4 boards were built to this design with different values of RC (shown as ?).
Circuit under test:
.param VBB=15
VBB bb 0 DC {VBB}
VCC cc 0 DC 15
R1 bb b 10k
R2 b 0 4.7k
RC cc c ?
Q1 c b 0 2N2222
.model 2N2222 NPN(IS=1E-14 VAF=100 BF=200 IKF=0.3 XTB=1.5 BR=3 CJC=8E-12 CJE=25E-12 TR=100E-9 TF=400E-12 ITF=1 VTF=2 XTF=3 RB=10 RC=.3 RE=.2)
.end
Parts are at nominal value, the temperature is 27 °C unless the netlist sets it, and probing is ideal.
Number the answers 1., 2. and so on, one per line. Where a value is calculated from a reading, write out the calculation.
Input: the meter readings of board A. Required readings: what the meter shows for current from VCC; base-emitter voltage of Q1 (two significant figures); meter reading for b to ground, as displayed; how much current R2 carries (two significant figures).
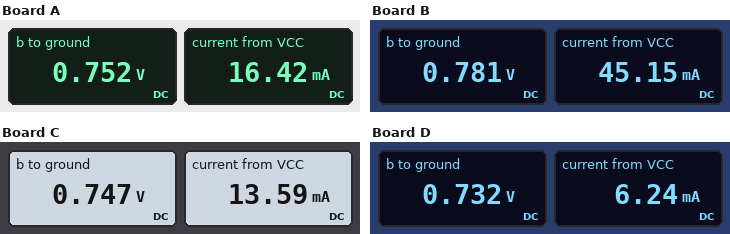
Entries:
1. 16.42 mA
2. 752 mV = 750 mV
3. 0.752 V
4. (752 mV) / 4.7 kΩ = 160 µA
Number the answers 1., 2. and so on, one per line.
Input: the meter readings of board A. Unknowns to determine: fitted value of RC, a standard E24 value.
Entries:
1. 910 Ω
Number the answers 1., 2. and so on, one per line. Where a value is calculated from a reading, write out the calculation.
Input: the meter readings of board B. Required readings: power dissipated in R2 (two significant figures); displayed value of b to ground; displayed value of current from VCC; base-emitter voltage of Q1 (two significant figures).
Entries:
1. (781 mV)^2 / 4.7 kΩ = 130 µW
2. 0.781 V
3. 45.15 mA
4. 781 mV = 780 mV
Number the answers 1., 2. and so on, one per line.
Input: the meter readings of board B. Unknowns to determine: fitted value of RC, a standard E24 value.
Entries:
1. 330 Ω
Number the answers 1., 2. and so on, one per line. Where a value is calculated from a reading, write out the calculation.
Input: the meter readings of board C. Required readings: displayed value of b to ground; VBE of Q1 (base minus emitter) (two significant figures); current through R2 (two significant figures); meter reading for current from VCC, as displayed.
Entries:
1. 0.747 V
2. 747 mV = 750 mV
3. (747 mV) / 4.7 kΩ = 160 µA
4. 13.59 mA
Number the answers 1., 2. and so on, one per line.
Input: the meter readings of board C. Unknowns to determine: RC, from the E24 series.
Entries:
1. 1.1 kΩ
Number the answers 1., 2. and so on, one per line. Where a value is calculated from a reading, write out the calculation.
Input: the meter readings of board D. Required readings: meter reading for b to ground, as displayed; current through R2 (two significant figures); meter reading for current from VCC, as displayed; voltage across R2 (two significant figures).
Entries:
1. 0.732 V
2. (732 mV) / 4.7 kΩ = 160 µA
3. 6.24 mA
4. 732 mV = 730 mV
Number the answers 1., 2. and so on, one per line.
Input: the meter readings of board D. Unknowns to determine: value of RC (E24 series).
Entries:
1. 2.4 kΩ
